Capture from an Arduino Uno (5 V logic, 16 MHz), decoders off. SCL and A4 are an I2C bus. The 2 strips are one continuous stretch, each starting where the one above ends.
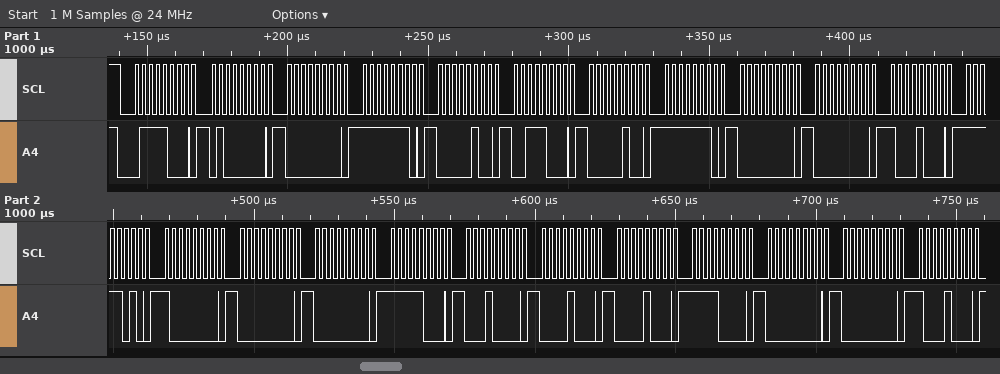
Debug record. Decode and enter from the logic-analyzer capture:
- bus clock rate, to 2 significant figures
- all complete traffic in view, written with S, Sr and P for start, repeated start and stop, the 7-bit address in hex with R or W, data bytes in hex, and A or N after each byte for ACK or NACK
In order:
400 kHz
S 3CW A 40 A 00 A FE A 04 A 38 A 04 A FE A 00 A 00 A 88 A FA A 80 A 00 A 00 A F8 A 10 A 08 A 08 A F0 A 00 A 00 A 88 A
